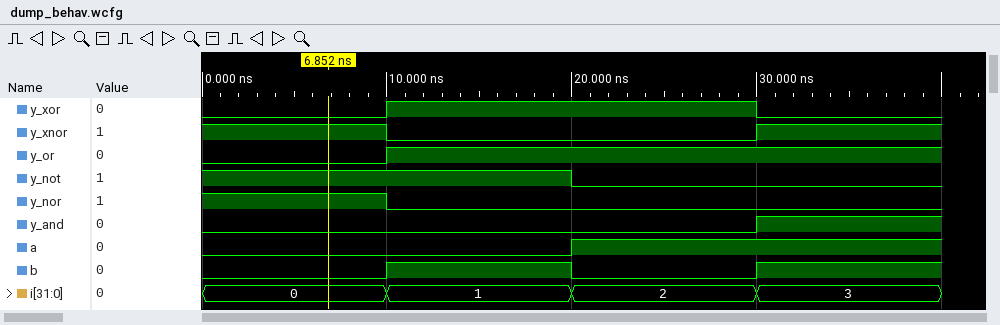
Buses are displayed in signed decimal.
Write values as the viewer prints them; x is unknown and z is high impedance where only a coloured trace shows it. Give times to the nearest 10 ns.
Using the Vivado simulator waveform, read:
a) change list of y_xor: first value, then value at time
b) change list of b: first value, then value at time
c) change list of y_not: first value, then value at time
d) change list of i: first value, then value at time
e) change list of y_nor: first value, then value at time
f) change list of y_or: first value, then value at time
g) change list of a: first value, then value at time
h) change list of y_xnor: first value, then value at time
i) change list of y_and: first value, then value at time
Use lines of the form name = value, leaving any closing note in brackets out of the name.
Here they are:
change list of y_xor: first value, then value at time = 0, 1 at 10 ns, 0 at 30 ns
change list of b: first value, then value at time = 0, 1 at 10 ns, 0 at 20 ns, 1 at 30 ns
change list of y_not: first value, then value at time = 1, 0 at 20 ns
change list of i: first value, then value at time = 0, 1 at 10 ns, 2 at 20 ns, 3 at 30 ns
change list of y_nor: first value, then value at time = 1, 0 at 10 ns
change list of y_or: first value, then value at time = 0, 1 at 10 ns
change list of a: first value, then value at time = 0, 1 at 20 ns
change list of y_xnor: first value, then value at time = 1, 0 at 10 ns, 1 at 30 ns
change list of y_and: first value, then value at time = 0, 1 at 30 ns
